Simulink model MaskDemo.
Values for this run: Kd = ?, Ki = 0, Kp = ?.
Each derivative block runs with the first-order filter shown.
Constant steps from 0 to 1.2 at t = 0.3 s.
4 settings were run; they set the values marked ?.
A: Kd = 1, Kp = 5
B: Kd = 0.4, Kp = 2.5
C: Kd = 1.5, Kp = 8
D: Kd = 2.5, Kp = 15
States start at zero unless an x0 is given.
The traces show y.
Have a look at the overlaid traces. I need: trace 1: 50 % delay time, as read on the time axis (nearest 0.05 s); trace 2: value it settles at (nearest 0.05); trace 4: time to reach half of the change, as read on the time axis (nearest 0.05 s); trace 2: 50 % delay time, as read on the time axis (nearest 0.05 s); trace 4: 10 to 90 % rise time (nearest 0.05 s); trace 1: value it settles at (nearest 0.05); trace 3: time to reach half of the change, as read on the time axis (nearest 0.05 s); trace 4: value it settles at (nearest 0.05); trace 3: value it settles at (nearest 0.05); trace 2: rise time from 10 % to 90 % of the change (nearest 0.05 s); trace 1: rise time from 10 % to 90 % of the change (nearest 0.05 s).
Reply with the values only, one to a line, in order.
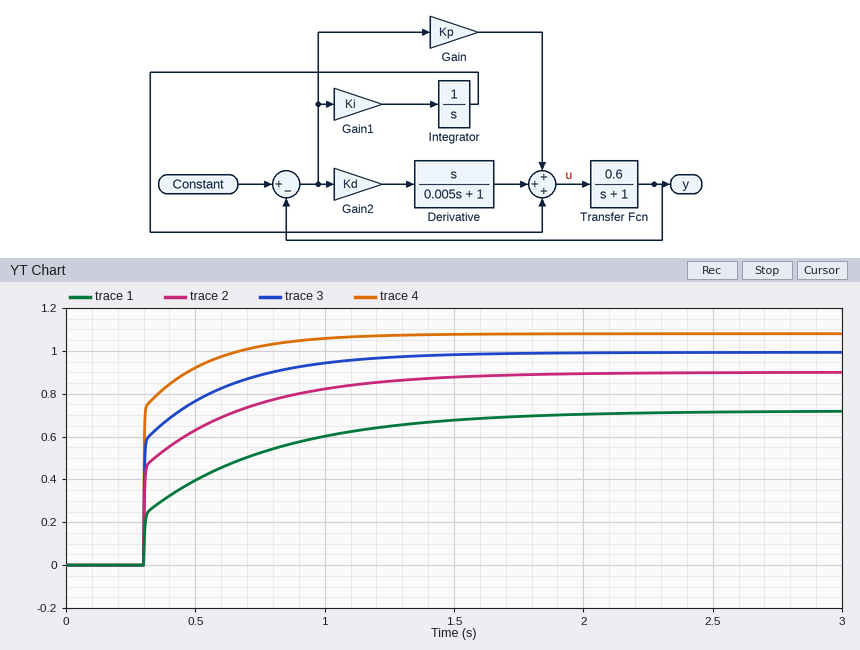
0.45 s
0.90
0.30 s
0.30 s
0.30 s
0.70
0.30 s
1.10
1.00
0.65 s
0.95 s
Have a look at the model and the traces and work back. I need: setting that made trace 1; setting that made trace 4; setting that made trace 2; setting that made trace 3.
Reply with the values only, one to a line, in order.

B
D
A
C
